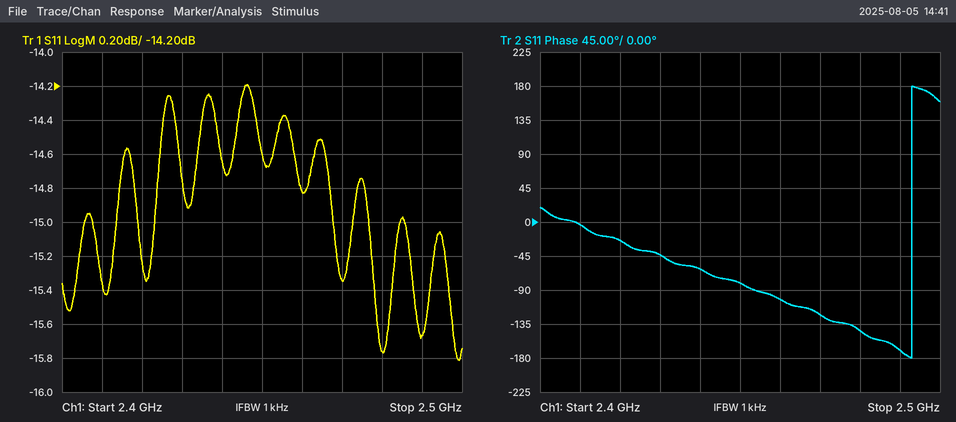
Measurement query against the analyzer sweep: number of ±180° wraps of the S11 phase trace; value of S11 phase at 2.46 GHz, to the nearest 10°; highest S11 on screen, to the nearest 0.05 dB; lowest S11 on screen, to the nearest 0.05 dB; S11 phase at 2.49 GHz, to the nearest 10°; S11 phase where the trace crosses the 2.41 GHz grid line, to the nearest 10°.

1
-100°
-14.20 dB
-15.80 dB
-170°
0°
